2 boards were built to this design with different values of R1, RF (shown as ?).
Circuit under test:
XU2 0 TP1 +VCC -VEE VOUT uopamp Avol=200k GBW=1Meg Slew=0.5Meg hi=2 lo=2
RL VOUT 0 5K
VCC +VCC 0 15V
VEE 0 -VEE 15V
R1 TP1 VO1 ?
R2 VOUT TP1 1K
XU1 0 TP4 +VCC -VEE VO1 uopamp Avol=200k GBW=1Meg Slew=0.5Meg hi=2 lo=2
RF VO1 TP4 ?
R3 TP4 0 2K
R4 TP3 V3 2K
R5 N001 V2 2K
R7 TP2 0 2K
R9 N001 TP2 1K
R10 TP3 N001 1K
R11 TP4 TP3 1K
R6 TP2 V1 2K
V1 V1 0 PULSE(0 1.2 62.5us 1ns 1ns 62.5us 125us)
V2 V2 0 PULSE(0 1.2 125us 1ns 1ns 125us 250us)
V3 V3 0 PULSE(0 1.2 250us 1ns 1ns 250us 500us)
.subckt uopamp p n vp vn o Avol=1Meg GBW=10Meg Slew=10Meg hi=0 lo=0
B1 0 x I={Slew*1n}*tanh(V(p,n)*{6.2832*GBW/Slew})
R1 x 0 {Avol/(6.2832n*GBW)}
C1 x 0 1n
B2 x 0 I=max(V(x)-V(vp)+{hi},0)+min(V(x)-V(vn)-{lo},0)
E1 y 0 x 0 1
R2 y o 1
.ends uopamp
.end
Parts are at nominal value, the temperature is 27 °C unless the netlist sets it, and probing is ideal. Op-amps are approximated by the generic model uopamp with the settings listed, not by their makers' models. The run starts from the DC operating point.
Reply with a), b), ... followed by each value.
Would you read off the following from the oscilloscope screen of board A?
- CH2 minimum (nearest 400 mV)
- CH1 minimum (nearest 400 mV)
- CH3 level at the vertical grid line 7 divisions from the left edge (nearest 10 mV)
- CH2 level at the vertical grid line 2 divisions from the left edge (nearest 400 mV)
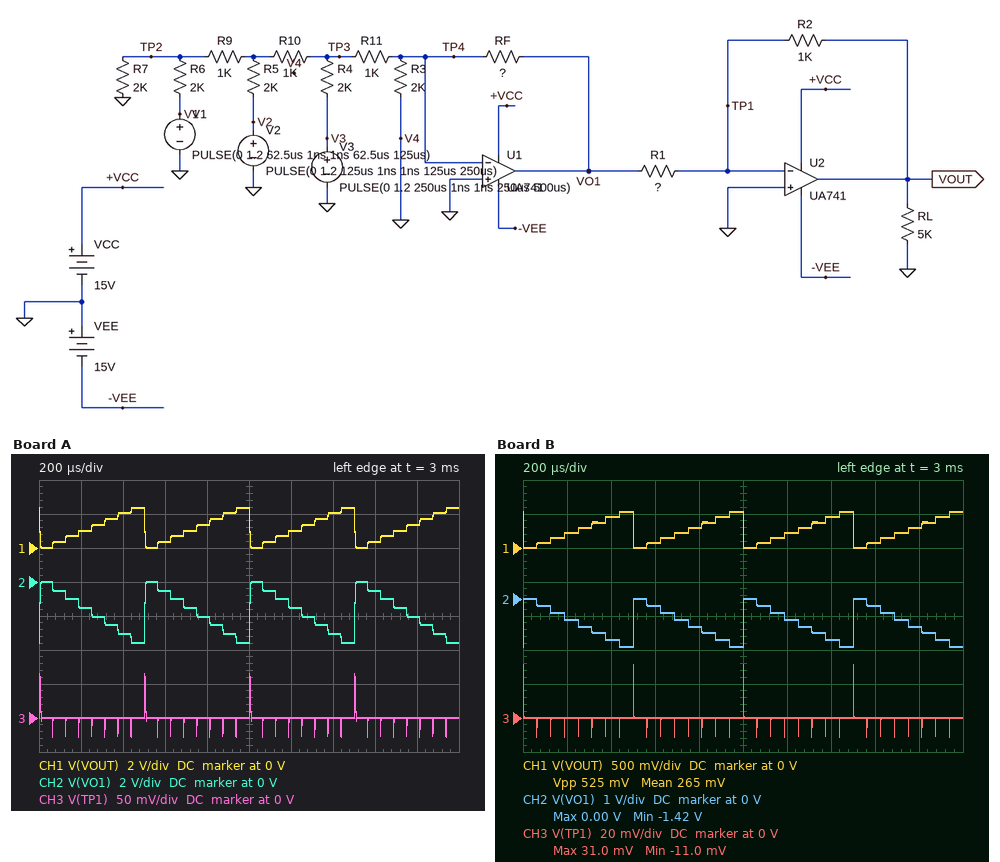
a) -3.6 V
b) 0 V
c) 0 V
d) -3.2 V
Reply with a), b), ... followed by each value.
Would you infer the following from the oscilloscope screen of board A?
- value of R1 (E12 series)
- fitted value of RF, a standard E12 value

a) 1.5 kΩ
b) 6.8 kΩ
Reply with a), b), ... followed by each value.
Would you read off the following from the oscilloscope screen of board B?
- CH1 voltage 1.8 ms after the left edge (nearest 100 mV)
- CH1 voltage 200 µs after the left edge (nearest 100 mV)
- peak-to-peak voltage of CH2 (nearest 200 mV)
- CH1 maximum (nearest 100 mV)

a) 300 mV
b) 200 mV
c) 1.4 V
d) 500 mV
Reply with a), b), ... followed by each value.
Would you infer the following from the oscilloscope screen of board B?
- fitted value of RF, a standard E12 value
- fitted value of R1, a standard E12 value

a) 2.7 kΩ
b) 2.7 kΩ
